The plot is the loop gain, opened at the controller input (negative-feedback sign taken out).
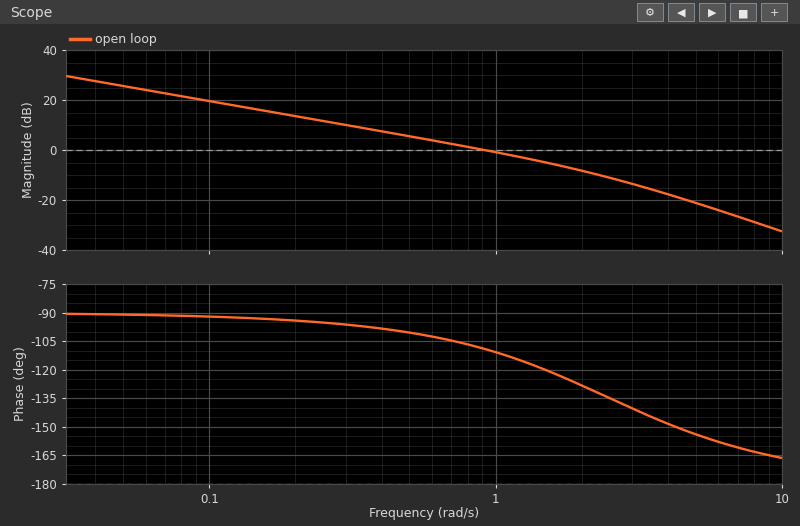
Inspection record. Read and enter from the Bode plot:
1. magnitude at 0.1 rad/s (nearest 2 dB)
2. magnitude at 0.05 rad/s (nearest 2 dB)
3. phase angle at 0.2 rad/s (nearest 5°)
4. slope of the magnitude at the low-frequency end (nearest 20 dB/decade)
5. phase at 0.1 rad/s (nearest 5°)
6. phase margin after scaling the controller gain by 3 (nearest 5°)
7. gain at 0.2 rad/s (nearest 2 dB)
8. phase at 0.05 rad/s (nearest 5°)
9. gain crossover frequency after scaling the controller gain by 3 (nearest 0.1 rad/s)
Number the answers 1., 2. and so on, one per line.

1. 20 dB
2. 26 dB
3. -95°
4. -20 dB/decade
5. -90°
6. 50°
7. 14 dB
8. -90°
9. 2.2 rad/s
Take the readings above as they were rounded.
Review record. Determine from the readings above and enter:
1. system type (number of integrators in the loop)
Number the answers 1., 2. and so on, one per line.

1. 1
